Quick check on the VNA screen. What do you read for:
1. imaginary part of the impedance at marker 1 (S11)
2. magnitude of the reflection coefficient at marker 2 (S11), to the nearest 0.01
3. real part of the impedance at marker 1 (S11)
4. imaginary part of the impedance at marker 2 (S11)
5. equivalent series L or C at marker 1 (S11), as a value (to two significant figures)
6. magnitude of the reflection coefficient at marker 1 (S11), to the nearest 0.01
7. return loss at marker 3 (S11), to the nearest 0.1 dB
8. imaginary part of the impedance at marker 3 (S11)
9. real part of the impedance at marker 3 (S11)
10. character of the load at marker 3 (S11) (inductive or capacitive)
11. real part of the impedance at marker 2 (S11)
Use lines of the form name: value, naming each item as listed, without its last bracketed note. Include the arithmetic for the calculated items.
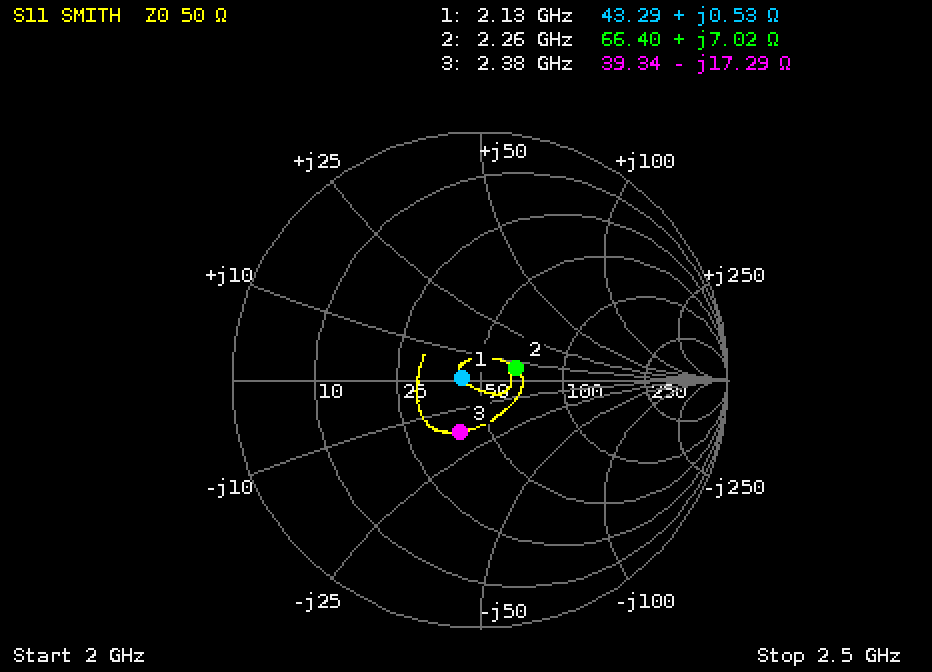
imaginary part of the impedance at marker 1: +0.53 Ω
magnitude of the reflection coefficient at marker 2 (S11), to the nearest 0.01: 0.15
real part of the impedance at marker 1: 43.29 Ω
imaginary part of the impedance at marker 2: +7.02 Ω
equivalent series L or C at marker 1 (S11), as a value: L = 0.53 Ω/(2π × 2.13 GHz) ≈ 40 pH
magnitude of the reflection coefficient at marker 1 (S11), to the nearest 0.01: 0.07
return loss at marker 3 (S11), to the nearest 0.1 dB: 13.0 dB
imaginary part of the impedance at marker 3: -17.29 Ω
real part of the impedance at marker 3: 39.34 Ω
character of the load at marker 3 (S11): capacitive
real part of the impedance at marker 2: 66.40 Ω
